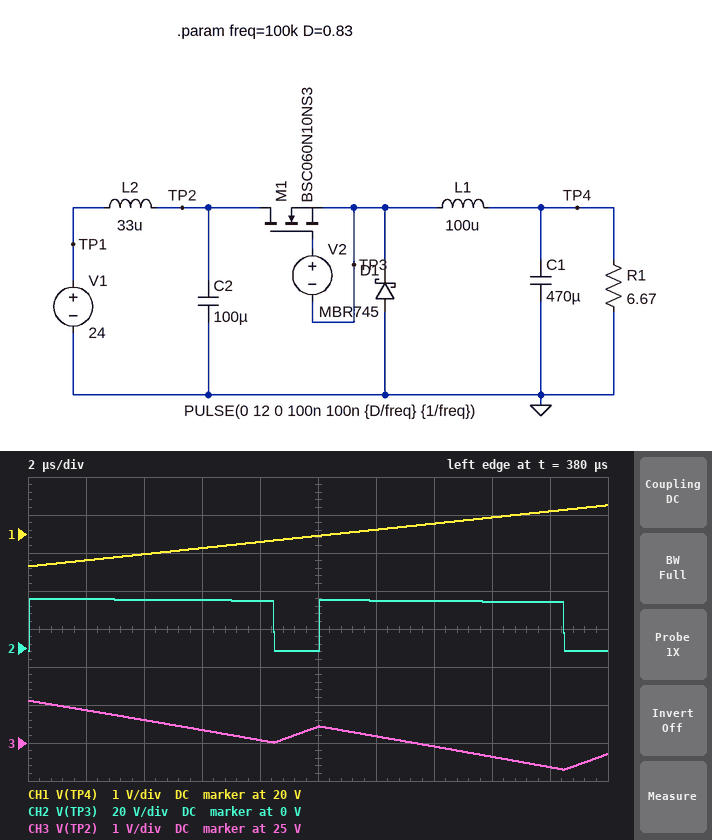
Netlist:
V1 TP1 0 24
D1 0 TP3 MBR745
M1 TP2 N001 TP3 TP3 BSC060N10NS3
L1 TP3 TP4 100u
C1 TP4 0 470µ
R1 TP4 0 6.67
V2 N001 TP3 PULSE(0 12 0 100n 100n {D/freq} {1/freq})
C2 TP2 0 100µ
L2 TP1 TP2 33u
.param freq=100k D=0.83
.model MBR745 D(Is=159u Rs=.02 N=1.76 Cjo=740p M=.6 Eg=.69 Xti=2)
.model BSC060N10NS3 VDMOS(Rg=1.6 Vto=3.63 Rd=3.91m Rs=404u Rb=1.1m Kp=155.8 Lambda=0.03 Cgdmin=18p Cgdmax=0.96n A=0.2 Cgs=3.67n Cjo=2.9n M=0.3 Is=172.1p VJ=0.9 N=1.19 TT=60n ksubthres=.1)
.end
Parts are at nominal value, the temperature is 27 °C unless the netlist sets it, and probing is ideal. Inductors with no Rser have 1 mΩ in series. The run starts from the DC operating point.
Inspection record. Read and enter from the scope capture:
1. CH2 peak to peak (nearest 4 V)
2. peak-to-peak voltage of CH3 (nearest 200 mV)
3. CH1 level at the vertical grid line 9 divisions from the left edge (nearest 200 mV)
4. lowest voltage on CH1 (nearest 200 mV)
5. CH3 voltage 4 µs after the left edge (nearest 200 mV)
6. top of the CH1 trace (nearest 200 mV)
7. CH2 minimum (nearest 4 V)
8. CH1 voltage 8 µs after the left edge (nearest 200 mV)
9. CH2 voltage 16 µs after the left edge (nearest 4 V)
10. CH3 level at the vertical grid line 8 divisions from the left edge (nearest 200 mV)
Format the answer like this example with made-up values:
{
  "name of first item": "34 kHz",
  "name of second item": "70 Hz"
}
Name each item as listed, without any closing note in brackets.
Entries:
{
  "CH2 peak to peak": "28 V",
  "peak-to-peak voltage of CH3": "1.8 V",
  "CH1 level at the vertical grid line 9 divisions from the left edge": "20.6 V",
  "lowest voltage on CH1": "19.2 V",
  "CH3 voltage 4 µs after the left edge": "25.6 V",
  "top of the CH1 trace": "20.8 V",
  "CH2 minimum": "0 V",
  "CH1 voltage 8 µs after the left edge": "19.8 V",
  "CH2 voltage 16 µs after the left edge": "24 V",
  "CH3 level at the vertical grid line 8 divisions from the left edge": "24.6 V"
}
